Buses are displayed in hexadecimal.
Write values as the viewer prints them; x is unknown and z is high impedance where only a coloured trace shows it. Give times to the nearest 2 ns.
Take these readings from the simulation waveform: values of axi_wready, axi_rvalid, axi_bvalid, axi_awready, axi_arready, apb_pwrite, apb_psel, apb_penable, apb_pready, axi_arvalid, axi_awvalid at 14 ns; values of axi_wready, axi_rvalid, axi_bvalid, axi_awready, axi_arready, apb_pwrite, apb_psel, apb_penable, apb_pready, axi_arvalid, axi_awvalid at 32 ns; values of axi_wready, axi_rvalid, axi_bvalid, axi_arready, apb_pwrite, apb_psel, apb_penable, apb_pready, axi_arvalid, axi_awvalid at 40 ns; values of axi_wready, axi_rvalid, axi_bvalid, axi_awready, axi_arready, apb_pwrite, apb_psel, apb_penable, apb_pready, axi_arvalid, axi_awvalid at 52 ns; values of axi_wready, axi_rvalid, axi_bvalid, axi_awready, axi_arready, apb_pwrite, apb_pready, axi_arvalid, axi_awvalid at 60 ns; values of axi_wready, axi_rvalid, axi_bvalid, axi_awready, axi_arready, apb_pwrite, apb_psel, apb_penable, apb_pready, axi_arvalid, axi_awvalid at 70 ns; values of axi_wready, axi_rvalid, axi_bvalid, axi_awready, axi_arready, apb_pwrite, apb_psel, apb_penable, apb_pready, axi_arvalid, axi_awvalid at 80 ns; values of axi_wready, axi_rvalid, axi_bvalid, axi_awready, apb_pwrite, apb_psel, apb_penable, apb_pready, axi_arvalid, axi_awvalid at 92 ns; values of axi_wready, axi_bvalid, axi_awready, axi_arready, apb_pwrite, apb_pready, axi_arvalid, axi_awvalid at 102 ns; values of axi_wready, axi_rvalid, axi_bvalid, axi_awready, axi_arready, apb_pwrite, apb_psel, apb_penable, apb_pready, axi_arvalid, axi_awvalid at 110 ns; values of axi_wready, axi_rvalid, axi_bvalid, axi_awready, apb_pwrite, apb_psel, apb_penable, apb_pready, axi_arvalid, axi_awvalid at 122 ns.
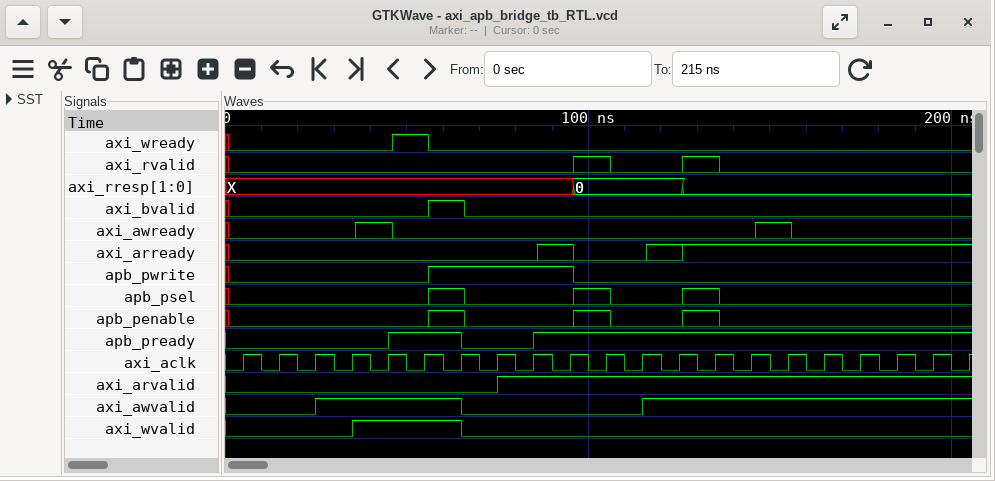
axi_wready=0, axi_rvalid=0, axi_bvalid=0, axi_awready=0, axi_arready=0, apb_pwrite=0, apb_psel=0, apb_penable=0, apb_pready=0, axi_arvalid=0, axi_awvalid=0
axi_wready=0, axi_rvalid=0, axi_bvalid=0, axi_awready=0, axi_arready=0, apb_pwrite=0, apb_psel=0, apb_penable=0, apb_pready=0, axi_arvalid=0, axi_awvalid=1
axi_wready=0, axi_rvalid=0, axi_bvalid=0, axi_arready=0, apb_pwrite=0, apb_psel=0, apb_penable=0, apb_pready=0, axi_arvalid=0, axi_awvalid=1
axi_wready=1, axi_rvalid=0, axi_bvalid=0, axi_awready=0, axi_arready=0, apb_pwrite=0, apb_psel=0, apb_penable=0, apb_pready=1, axi_arvalid=0, axi_awvalid=1
axi_wready=0, axi_rvalid=0, axi_bvalid=1, axi_awready=0, axi_arready=0, apb_pwrite=1, apb_pready=1, axi_arvalid=0, axi_awvalid=1
axi_wready=0, axi_rvalid=0, axi_bvalid=0, axi_awready=0, axi_arready=0, apb_pwrite=1, apb_psel=0, apb_penable=0, apb_pready=0, axi_arvalid=0, axi_awvalid=0
axi_wready=0, axi_rvalid=0, axi_bvalid=0, axi_awready=0, axi_arready=0, apb_pwrite=1, apb_psel=0, apb_penable=0, apb_pready=0, axi_arvalid=1, axi_awvalid=0
axi_wready=0, axi_rvalid=0, axi_bvalid=0, axi_awready=0, apb_pwrite=1, apb_psel=0, apb_penable=0, apb_pready=1, axi_arvalid=1, axi_awvalid=0
axi_wready=0, axi_bvalid=0, axi_awready=0, axi_arready=0, apb_pwrite=0, apb_pready=1, axi_arvalid=1, axi_awvalid=0
axi_wready=0, axi_rvalid=0, axi_bvalid=0, axi_awready=0, axi_arready=0, apb_pwrite=0, apb_psel=0, apb_penable=0, apb_pready=1, axi_arvalid=1, axi_awvalid=0
axi_wready=0, axi_rvalid=0, axi_bvalid=0, axi_awready=0, apb_pwrite=0, apb_psel=0, apb_penable=0, apb_pready=1, axi_arvalid=1, axi_awvalid=1
